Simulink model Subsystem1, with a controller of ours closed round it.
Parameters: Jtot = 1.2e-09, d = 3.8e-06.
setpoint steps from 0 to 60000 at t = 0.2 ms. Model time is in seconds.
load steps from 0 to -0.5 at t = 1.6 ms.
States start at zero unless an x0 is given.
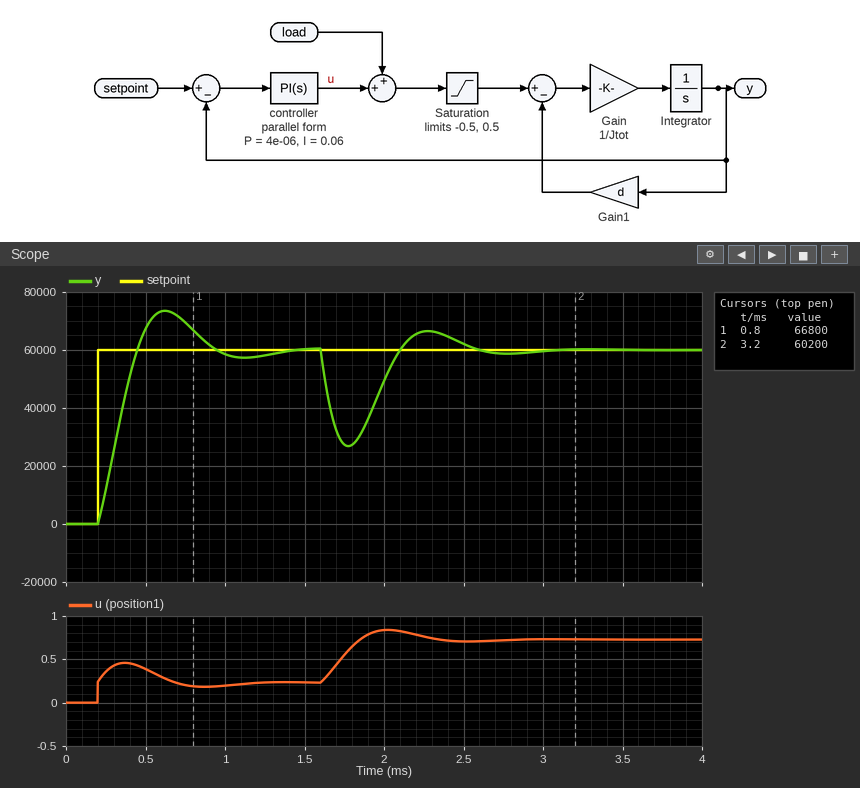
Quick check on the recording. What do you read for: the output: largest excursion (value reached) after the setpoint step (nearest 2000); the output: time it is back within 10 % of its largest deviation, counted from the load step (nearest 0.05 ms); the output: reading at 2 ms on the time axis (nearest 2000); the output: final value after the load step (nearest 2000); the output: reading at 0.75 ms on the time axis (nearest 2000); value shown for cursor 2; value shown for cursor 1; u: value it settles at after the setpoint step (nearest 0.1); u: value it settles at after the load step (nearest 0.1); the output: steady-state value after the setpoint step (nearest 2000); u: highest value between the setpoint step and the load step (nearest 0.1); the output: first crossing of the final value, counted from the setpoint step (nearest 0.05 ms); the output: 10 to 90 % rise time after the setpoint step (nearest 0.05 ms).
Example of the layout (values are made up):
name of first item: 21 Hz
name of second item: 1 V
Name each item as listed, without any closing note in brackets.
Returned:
the output: largest excursion (value reached) after the setpoint step: 74000
the output: time it is back within 10 % of its largest deviation, counted from the load step: 0.85 ms
the output: reading at 2 ms on the time axis: 50000
the output: final value after the load step: 60000
the output: reading at 0.75 ms on the time axis: 70000
value shown for cursor 2: 60200
value shown for cursor 1: 66800
u: value it settles at after the setpoint step: 0.2
u: value it settles at after the load step: 0.7
the output: steady-state value after the setpoint step: 60000
u: highest value between the setpoint step and the load step: 0.5
the output: first crossing of the final value, counted from the setpoint step: 0.25 ms
the output: 10 to 90 % rise time after the setpoint step: 0.20 ms
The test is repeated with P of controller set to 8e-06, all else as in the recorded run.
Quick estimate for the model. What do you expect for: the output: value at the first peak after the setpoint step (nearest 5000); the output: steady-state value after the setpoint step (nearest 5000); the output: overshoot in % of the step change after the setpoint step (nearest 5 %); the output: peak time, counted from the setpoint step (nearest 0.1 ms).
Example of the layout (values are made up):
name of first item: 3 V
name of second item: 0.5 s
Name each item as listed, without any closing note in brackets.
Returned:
the output: value at the first peak after the setpoint step: 65000
the output: steady-state value after the setpoint step: 60000
the output: overshoot in % of the step change after the setpoint step: 10 %
the output: peak time, counted from the setpoint step: 0.4 ms
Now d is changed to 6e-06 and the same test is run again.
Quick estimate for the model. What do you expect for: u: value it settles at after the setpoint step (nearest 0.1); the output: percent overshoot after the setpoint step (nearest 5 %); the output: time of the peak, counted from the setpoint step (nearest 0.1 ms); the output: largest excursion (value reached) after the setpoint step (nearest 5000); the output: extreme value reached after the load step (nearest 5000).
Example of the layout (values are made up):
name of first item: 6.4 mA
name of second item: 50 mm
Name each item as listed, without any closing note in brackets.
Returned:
u: value it settles at after the setpoint step: 0.4
the output: percent overshoot after the setpoint step: 10 %
the output: time of the peak, counted from the setpoint step: 0.5 ms
the output: largest excursion (value reached) after the setpoint step: 65000
the output: extreme value reached after the load step: 30000
